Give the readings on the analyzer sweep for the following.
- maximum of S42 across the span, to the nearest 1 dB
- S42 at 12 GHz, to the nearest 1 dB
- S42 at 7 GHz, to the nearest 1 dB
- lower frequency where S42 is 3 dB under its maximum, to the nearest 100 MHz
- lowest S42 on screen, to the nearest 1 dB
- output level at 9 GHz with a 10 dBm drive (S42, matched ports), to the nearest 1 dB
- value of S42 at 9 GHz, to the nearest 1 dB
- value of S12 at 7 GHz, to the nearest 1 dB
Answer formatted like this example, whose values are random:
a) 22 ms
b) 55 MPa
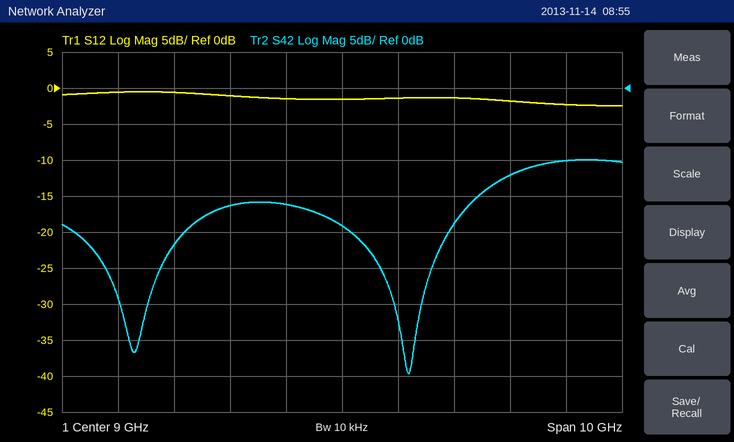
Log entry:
a) -10 dB
b) -12 dB
c) -16 dB
d) 11.8 GHz
e) -40 dB
f) -9 dBm
g) -19 dB
h) -1 dB
